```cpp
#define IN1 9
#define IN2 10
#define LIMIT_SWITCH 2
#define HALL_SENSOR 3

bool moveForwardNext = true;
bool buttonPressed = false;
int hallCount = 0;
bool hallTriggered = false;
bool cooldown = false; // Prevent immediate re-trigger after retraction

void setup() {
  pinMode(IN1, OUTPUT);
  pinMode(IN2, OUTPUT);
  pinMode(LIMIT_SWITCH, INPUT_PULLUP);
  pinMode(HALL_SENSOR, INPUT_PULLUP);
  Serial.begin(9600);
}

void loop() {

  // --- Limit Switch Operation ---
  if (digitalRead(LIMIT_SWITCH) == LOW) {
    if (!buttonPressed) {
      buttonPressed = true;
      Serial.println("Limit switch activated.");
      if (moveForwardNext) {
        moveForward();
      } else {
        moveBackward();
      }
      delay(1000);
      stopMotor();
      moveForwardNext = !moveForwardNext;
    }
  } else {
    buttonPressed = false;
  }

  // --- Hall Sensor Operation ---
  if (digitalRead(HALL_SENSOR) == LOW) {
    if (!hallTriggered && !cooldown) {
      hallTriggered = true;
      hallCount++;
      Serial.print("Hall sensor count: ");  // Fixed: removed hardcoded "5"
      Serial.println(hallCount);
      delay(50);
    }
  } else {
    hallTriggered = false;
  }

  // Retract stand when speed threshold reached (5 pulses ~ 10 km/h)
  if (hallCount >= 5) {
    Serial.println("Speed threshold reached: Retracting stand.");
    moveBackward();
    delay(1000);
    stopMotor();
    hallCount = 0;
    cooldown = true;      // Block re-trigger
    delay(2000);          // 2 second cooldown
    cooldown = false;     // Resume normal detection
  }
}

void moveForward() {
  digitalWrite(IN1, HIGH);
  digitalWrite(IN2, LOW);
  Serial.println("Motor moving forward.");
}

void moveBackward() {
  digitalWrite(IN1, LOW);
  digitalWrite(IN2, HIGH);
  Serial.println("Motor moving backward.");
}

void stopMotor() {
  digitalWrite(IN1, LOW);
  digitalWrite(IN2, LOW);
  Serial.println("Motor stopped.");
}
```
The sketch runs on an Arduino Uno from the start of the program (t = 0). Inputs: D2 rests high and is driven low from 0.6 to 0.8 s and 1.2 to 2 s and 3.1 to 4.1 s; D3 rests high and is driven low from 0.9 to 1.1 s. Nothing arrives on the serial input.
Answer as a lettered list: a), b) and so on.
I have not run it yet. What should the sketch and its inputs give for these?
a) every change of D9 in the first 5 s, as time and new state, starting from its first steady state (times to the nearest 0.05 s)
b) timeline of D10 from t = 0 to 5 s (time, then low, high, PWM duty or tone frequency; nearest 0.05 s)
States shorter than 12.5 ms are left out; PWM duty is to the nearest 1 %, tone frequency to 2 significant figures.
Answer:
a) 0 s low; 0.6 s high; 1.6 s low
b) 0 s low; 3.1 s high; 4.1 s low
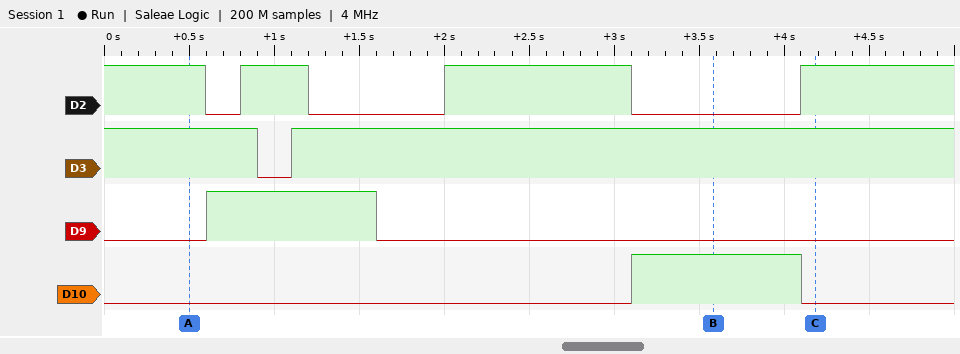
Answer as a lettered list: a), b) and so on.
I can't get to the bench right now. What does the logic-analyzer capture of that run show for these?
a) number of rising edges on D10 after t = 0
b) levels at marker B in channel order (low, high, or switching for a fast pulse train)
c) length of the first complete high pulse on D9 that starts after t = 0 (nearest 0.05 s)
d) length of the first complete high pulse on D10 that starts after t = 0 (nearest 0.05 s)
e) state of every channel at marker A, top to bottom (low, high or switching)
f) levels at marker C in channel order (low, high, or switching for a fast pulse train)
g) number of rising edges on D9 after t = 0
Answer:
a) 1
b) D2 low, D3 high, D9 low, D10 high
c) 1.00 s
d) 1.00 s
e) D2 high, D3 high, D9 low, D10 low
f) D2 high, D3 high, D9 low, D10 low
g) 1
